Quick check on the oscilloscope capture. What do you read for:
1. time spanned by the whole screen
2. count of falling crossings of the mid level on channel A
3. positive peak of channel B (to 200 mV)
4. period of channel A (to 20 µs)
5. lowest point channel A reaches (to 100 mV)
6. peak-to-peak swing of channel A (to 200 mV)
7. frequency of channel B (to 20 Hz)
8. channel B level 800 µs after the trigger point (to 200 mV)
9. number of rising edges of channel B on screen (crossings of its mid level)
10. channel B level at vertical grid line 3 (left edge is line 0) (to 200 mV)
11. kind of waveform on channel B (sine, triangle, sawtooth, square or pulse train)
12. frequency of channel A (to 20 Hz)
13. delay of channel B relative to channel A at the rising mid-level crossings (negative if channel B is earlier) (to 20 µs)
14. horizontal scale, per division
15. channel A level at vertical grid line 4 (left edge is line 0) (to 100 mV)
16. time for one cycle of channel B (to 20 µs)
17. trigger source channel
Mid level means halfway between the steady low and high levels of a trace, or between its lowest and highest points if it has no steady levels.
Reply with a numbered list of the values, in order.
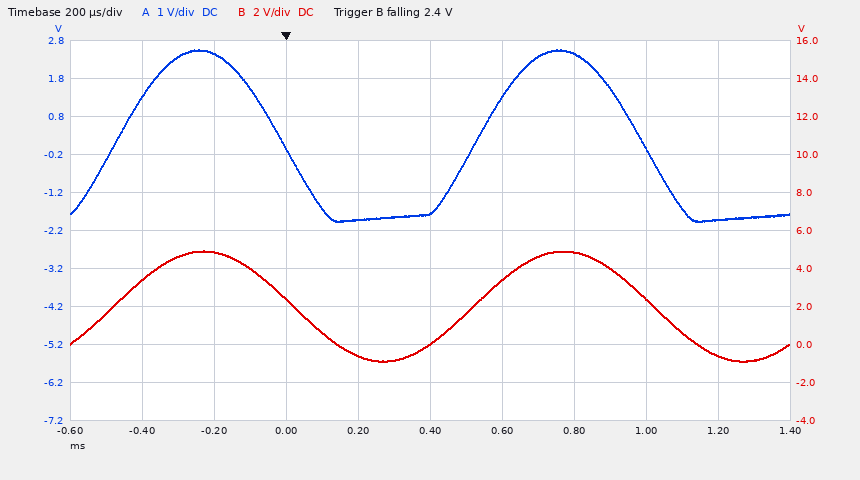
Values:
1. 2 ms
2. 2
3. 5.0 V
4. 1.00 ms
5. -2.0 V
6. 4.6 V
7. 1.00 kHz
8. 4.8 V
9. 2
10. 2.4 V
11. sine
12. 1.00 kHz
13. -20 µs
14. 200 µs
15. -1.9 V
16. 1.00 ms
17. channel B
